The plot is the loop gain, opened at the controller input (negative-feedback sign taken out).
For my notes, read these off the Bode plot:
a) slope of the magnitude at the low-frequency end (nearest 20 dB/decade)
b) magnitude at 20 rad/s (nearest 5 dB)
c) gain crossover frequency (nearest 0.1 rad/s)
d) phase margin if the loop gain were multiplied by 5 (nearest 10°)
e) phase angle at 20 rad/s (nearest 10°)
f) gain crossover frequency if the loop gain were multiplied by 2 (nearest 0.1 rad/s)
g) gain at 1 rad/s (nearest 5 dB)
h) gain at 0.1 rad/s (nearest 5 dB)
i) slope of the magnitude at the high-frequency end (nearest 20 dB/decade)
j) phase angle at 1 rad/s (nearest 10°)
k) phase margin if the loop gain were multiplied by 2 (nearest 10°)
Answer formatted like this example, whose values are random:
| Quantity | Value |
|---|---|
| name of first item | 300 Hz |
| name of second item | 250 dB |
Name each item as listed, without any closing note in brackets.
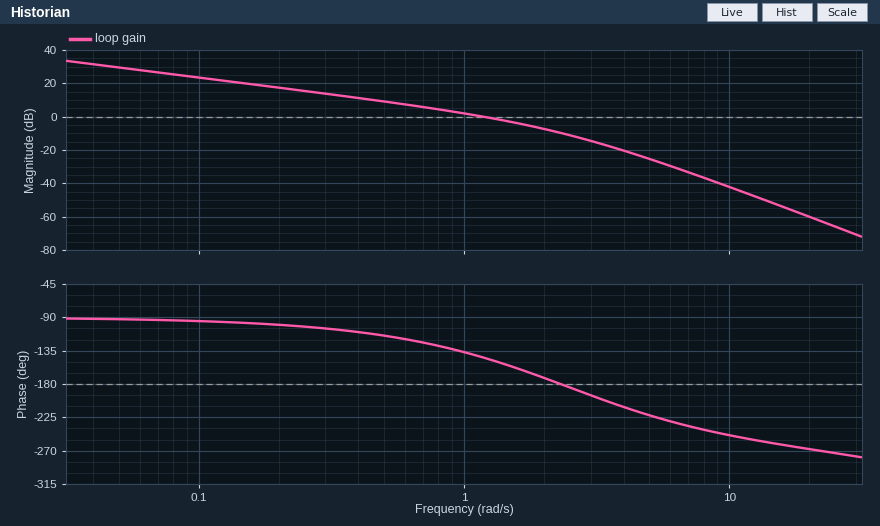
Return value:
| Quantity | Value |
|---|---|
| slope of the magnitude at the low-frequency end | -20 dB/decade |
| magnitude at 20 rad/s | -60 dB |
| gain crossover frequency | 1.2 rad/s |
| phase margin if the loop gain were multiplied by 5 | -10° |
| phase angle at 20 rad/s | -270° |
| gain crossover frequency if the loop gain were multiplied by 2 | 1.8 rad/s |
| gain at 1 rad/s | 0 dB |
| gain at 0.1 rad/s | 25 dB |
| slope of the magnitude at the high-frequency end | -60 dB/decade |
| phase angle at 1 rad/s | -140° |
| phase margin if the loop gain were multiplied by 2 | 10° |
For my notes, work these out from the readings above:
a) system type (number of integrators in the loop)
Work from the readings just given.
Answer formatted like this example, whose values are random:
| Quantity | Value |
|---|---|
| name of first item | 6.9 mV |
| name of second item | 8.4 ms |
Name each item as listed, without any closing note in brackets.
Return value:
| Quantity | Value |
|---|---|
| system type | 1 |
